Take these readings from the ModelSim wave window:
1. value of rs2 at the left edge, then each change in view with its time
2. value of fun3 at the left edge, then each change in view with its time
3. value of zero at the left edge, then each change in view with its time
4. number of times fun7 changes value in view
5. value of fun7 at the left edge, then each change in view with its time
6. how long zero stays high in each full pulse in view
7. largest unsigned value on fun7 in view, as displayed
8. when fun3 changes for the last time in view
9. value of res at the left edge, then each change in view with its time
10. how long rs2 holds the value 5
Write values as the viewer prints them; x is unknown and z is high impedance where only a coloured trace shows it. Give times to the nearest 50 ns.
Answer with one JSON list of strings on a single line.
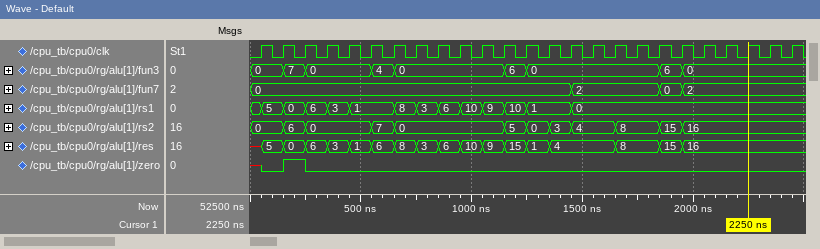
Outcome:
["0, 6 at 150 ns, 0 at 250 ns, 7 at 550 ns, 0 at 650 ns, 5 at 1150 ns, 0 at 1250 ns, 3 at 1350 ns, 4 at 1450 ns, 8 at 1650 ns, 15 at 1850 ns, 16 at 1950 ns", "0, 7 at 150 ns, 0 at 250 ns, 4 at 550 ns, 0 at 650 ns, 6 at 1150 ns, 0 at 1250 ns, 6 at 1850 ns, 0 at 1950 ns", "x, 0 at 50 ns, 1 at 150 ns, 0 at 250 ns", "3", "0, 2 at 1450 ns, 0 at 1850 ns, 2 at 1950 ns", "100 ns", "2", "1950 ns", "x, 5 at 50 ns, 0 at 150 ns, 6 at 250 ns, 3 at 350 ns, 1 at 450 ns, 6 at 550 ns, 8 at 650 ns, 3 at 750 ns, 6 at 850 ns, 10 at 950 ns, 9 at 1050 ns, 15 at 1150 ns, 1 at 1250 ns, 4 at 1350 ns, 8 at 1650 ns, 15 at 1850 ns, 16 at 1950 ns", "100 ns"]
